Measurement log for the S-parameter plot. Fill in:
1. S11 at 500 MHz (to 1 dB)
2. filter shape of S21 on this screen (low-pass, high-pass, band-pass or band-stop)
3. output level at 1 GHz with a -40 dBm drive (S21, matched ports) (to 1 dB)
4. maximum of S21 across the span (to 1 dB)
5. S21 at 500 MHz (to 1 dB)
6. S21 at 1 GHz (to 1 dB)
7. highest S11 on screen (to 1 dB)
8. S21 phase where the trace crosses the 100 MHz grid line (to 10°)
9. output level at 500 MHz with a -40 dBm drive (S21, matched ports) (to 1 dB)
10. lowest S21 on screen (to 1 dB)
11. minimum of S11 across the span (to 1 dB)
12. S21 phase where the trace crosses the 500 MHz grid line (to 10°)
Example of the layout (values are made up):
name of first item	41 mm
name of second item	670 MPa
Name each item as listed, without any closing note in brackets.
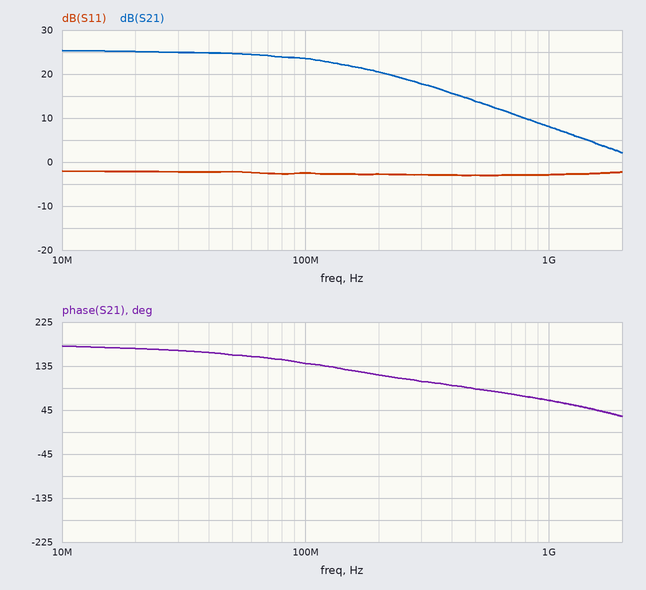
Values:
S11 at 500 MHz	-3 dB
filter shape of S21 on this screen	low-pass
output level at 1 GHz with a -40 dBm drive (S21, matched ports)	-32 dBm
maximum of S21 across the span	25 dB
S21 at 500 MHz	14 dB
S21 at 1 GHz	8 dB
highest S11 on screen	-2 dB
S21 phase where the trace crosses the 100 MHz grid line	140°
output level at 500 MHz with a -40 dBm drive (S21, matched ports)	-26 dBm
lowest S21 on screen	2 dB
minimum of S11 across the span	-3 dB
S21 phase where the trace crosses the 500 MHz grid line	90°
